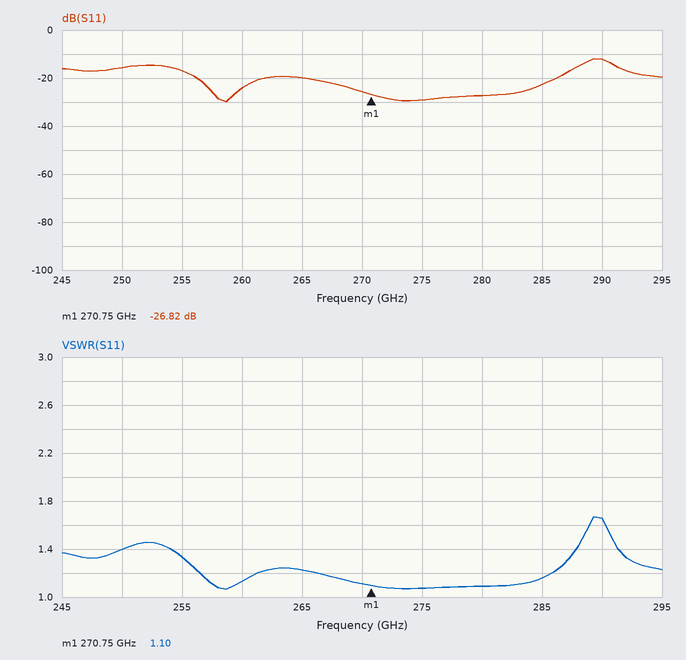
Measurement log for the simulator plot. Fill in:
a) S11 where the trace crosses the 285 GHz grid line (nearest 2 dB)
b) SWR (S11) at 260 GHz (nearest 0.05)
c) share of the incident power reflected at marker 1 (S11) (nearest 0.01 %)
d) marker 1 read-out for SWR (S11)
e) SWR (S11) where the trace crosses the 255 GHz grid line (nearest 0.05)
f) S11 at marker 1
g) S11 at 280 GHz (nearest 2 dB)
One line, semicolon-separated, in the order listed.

-22 dB; 1.15; 0.21 %; 1.10; 1.35; -26.82 dB; -28 dB
